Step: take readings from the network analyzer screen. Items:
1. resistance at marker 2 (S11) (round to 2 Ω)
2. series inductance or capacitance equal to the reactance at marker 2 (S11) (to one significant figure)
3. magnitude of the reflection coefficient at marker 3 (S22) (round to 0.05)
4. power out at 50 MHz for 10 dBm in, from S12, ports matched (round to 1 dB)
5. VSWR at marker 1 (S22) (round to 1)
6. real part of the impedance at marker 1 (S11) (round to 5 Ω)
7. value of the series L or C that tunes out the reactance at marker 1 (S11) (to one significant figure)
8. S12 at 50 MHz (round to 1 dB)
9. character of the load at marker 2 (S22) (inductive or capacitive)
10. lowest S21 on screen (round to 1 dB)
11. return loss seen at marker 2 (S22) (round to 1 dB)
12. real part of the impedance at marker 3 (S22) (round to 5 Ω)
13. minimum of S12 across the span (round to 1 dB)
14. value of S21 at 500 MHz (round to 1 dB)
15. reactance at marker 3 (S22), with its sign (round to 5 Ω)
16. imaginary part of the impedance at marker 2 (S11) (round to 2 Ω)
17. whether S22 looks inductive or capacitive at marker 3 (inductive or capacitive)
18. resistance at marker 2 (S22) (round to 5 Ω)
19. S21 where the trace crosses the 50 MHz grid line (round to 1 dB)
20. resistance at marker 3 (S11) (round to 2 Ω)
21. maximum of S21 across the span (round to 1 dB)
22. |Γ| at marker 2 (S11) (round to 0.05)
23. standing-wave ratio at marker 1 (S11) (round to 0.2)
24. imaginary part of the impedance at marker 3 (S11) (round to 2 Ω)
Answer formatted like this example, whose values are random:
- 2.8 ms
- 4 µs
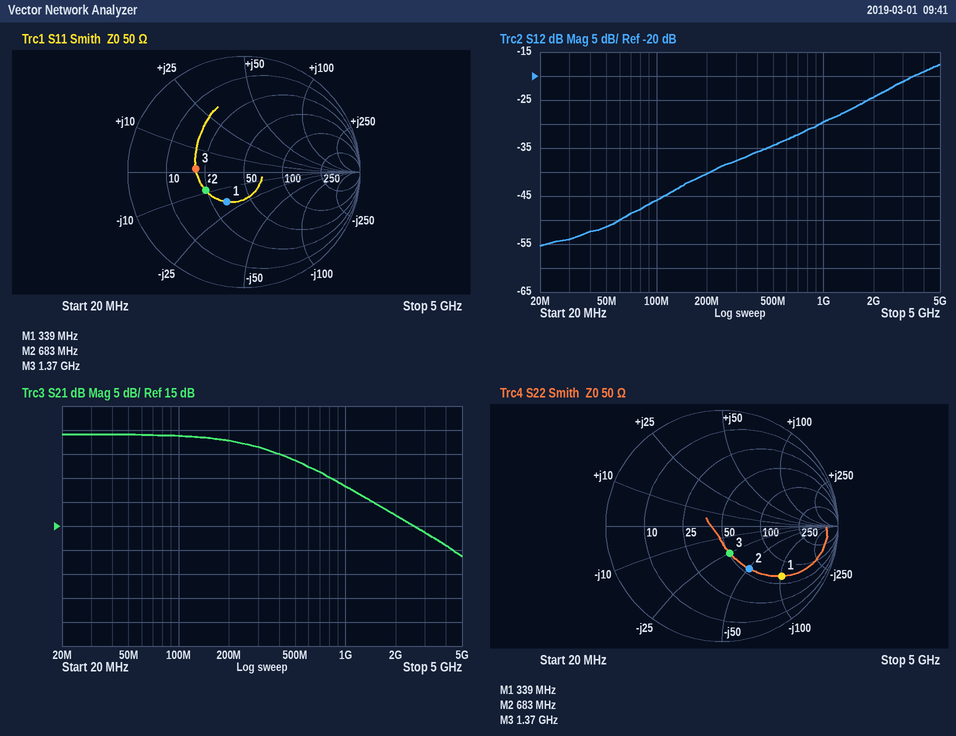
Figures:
- 24 Ω
- 30 pF
- 0.25
- -41 dBm
- 5
- 35 Ω
- 9 nH
- -51 dB
- capacitive
- 9 dB
- 7 dB
- 50 Ω
- -55 dB
- 29 dB
- -25 Ω
- -8 Ω
- capacitive
- 55 Ω
- 34 dB
- 20 Ω
- 34 dB
- 0.35
- 1.8
- +2 Ω
